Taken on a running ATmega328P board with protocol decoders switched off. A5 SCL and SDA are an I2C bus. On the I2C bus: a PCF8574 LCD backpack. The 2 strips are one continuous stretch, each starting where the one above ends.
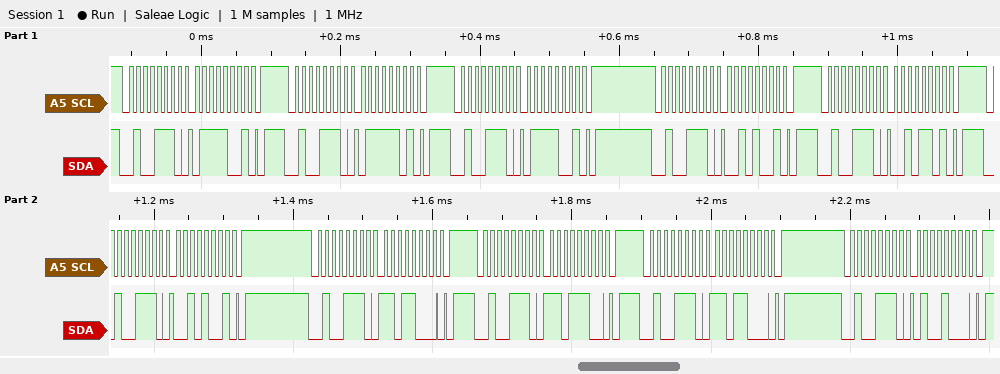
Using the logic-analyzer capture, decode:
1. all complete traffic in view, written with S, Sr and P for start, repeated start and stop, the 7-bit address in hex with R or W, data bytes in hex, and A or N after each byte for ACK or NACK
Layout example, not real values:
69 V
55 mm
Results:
S 27W A 79 A P S 27W A 7D A P S 27W A 79 A P S 27W A 29 A P S 27W A 2D A P S 27W A 29 A P S 27W A D8 A P S 27W A DC A P S 27W A D8 A P S 27W A 48 A P
